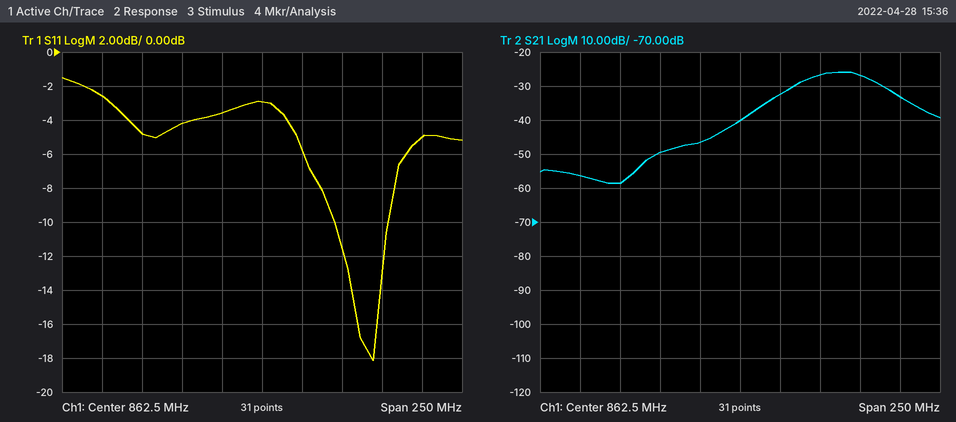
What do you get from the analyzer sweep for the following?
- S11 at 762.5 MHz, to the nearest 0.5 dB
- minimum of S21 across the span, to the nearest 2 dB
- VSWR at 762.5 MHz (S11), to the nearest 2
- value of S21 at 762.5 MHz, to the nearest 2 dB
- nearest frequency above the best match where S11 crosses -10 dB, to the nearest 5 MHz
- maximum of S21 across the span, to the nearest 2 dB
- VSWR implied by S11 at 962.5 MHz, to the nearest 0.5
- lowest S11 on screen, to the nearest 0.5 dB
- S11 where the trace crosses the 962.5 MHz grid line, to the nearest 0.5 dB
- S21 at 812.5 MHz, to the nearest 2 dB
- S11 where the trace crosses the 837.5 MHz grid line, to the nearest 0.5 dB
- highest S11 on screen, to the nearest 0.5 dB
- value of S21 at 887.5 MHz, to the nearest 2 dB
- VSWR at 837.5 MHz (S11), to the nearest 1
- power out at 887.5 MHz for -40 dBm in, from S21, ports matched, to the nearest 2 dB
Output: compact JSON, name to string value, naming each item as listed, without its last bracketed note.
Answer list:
{"S11 at 762.5 MHz, to the nearest 0.5 dB": "-2.5 dB", "minimum of S21 across the span, to the nearest 2 dB": "-58 dB", "VSWR at 762.5 MHz (S11), to the nearest 2": "6", "value of S21 at 762.5 MHz, to the nearest 2 dB": "-56 dB", "nearest frequency above the best match where S11 crosses -10 dB, to the nearest 5 MHz": "940 MHz", "maximum of S21 across the span, to the nearest 2 dB": "-26 dB", "VSWR implied by S11 at 962.5 MHz, to the nearest 0.5": "3.5", "lowest S11 on screen, to the nearest 0.5 dB": "-18.0 dB", "S11 where the trace crosses the 962.5 MHz grid line, to the nearest 0.5 dB": "-5.0 dB", "S21 at 812.5 MHz, to the nearest 2 dB": "-50 dB", "S11 where the trace crosses the 837.5 MHz grid line, to the nearest 0.5 dB": "-3.5 dB", "highest S11 on screen, to the nearest 0.5 dB": "-1.5 dB", "value of S21 at 887.5 MHz, to the nearest 2 dB": "-32 dB", "VSWR at 837.5 MHz (S11), to the nearest 1": "5", "power out at 887.5 MHz for -40 dBm in, from S21, ports matched, to the nearest 2 dB": "-72 dBm"}
